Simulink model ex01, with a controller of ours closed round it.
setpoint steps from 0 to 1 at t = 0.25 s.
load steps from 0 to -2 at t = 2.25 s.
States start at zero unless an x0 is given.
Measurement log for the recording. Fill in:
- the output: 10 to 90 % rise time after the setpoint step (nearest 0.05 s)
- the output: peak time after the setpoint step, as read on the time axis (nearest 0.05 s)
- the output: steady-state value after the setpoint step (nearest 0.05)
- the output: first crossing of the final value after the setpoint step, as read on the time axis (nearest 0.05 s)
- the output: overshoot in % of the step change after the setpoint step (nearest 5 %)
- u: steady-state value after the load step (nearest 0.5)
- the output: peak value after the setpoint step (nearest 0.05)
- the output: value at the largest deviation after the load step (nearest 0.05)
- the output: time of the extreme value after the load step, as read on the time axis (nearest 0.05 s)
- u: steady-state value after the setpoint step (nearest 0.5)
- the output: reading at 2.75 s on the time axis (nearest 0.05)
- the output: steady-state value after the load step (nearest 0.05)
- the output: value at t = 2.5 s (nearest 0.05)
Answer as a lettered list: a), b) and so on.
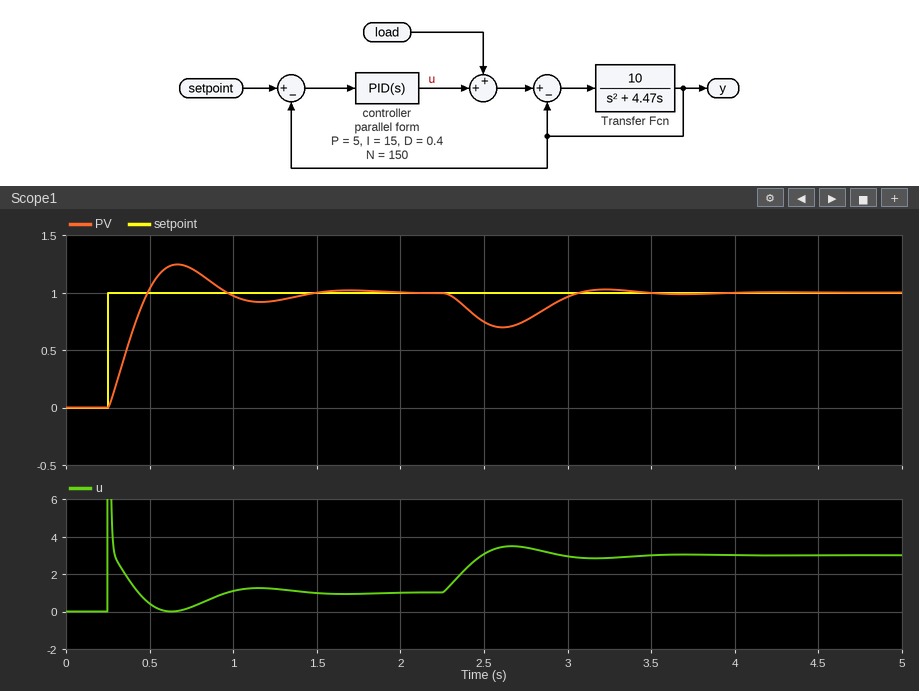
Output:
a) 0.20 s
b) 0.65 s
c) 1.00
d) 0.50 s
e) 25 %
f) 3.0
g) 1.25
h) 0.70
i) 2.60 s
j) 1.0
k) 0.75
l) 1.00
m) 0.75
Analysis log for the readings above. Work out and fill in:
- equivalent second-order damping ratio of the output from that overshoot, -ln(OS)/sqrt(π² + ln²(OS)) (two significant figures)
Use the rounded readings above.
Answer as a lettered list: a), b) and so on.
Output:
a) 0.40
